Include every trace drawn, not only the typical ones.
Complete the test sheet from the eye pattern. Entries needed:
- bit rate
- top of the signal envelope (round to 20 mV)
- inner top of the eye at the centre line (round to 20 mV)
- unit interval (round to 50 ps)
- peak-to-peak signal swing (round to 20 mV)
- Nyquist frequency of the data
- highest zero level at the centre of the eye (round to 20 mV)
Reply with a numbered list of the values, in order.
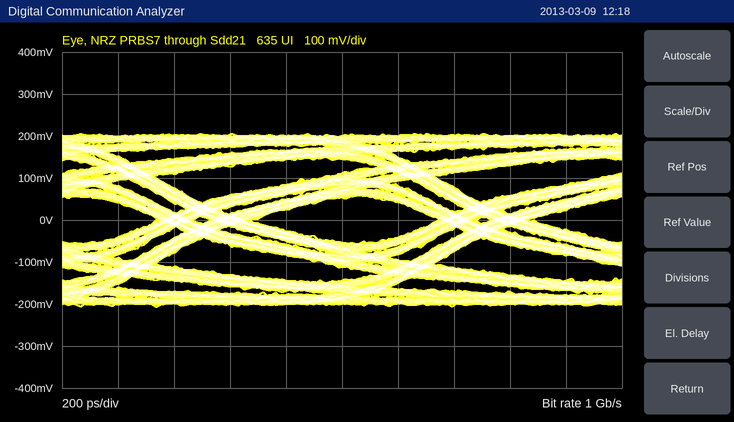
1. 1 Gb/s
2. 200 mV
3. 60 mV
4. 1.00 ns
5. 420 mV
6. 500 MHz
7. -60 mV
